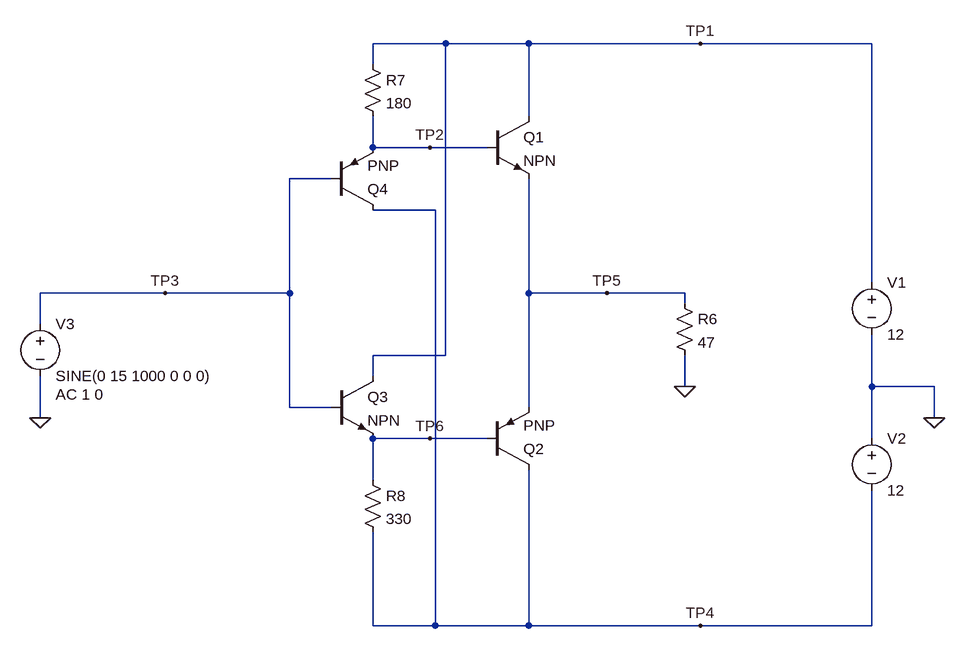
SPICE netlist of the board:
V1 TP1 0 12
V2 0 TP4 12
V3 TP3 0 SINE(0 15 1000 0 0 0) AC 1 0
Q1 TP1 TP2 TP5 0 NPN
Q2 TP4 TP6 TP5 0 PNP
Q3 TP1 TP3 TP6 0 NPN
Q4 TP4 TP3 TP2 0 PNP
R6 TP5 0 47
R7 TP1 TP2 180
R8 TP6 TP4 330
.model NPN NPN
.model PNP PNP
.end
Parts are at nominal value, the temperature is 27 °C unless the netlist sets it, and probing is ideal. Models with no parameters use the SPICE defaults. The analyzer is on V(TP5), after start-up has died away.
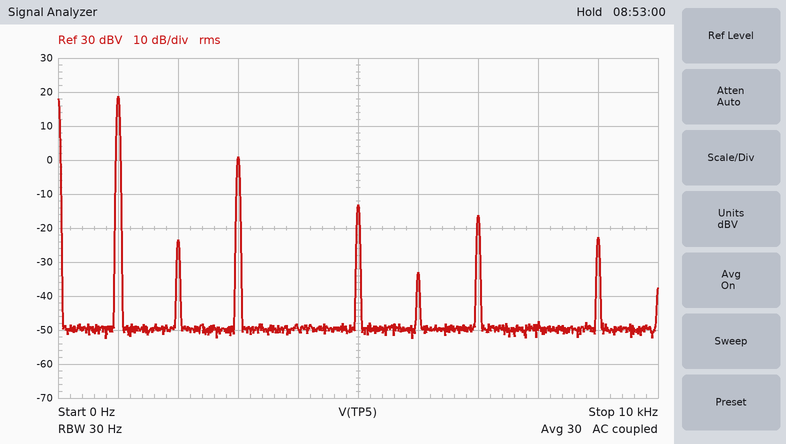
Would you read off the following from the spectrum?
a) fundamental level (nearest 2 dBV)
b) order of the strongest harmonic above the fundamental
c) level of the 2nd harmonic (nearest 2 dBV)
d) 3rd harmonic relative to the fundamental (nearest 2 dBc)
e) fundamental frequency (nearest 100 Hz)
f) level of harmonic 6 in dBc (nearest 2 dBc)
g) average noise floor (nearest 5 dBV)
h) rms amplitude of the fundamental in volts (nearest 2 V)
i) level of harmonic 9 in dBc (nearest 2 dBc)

18 dBV
3
-24 dBV
-18 dBc
1.0 kHz
-52 dBc
-50 dBV
8 V
-42 dBc
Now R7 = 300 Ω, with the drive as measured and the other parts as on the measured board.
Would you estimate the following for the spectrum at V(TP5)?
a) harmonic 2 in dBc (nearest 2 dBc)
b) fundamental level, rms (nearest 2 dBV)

-56 dBc
18 dBV
